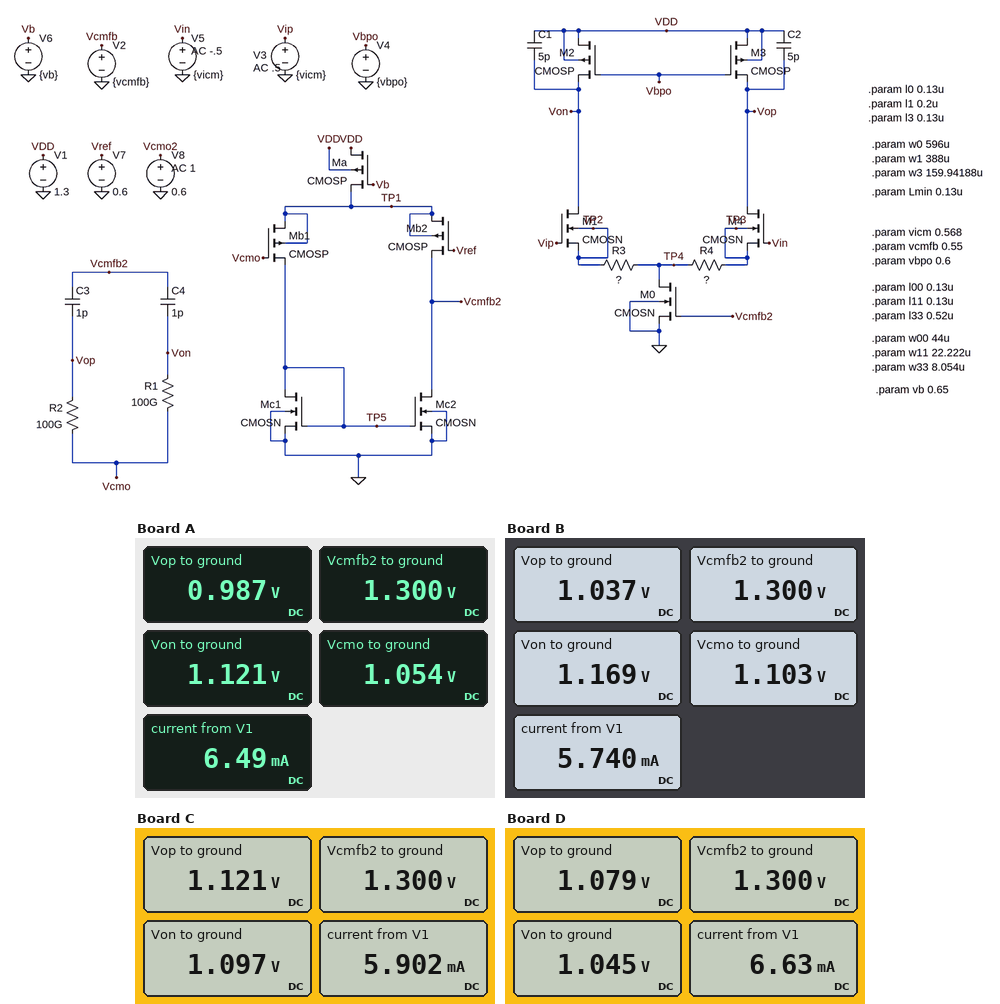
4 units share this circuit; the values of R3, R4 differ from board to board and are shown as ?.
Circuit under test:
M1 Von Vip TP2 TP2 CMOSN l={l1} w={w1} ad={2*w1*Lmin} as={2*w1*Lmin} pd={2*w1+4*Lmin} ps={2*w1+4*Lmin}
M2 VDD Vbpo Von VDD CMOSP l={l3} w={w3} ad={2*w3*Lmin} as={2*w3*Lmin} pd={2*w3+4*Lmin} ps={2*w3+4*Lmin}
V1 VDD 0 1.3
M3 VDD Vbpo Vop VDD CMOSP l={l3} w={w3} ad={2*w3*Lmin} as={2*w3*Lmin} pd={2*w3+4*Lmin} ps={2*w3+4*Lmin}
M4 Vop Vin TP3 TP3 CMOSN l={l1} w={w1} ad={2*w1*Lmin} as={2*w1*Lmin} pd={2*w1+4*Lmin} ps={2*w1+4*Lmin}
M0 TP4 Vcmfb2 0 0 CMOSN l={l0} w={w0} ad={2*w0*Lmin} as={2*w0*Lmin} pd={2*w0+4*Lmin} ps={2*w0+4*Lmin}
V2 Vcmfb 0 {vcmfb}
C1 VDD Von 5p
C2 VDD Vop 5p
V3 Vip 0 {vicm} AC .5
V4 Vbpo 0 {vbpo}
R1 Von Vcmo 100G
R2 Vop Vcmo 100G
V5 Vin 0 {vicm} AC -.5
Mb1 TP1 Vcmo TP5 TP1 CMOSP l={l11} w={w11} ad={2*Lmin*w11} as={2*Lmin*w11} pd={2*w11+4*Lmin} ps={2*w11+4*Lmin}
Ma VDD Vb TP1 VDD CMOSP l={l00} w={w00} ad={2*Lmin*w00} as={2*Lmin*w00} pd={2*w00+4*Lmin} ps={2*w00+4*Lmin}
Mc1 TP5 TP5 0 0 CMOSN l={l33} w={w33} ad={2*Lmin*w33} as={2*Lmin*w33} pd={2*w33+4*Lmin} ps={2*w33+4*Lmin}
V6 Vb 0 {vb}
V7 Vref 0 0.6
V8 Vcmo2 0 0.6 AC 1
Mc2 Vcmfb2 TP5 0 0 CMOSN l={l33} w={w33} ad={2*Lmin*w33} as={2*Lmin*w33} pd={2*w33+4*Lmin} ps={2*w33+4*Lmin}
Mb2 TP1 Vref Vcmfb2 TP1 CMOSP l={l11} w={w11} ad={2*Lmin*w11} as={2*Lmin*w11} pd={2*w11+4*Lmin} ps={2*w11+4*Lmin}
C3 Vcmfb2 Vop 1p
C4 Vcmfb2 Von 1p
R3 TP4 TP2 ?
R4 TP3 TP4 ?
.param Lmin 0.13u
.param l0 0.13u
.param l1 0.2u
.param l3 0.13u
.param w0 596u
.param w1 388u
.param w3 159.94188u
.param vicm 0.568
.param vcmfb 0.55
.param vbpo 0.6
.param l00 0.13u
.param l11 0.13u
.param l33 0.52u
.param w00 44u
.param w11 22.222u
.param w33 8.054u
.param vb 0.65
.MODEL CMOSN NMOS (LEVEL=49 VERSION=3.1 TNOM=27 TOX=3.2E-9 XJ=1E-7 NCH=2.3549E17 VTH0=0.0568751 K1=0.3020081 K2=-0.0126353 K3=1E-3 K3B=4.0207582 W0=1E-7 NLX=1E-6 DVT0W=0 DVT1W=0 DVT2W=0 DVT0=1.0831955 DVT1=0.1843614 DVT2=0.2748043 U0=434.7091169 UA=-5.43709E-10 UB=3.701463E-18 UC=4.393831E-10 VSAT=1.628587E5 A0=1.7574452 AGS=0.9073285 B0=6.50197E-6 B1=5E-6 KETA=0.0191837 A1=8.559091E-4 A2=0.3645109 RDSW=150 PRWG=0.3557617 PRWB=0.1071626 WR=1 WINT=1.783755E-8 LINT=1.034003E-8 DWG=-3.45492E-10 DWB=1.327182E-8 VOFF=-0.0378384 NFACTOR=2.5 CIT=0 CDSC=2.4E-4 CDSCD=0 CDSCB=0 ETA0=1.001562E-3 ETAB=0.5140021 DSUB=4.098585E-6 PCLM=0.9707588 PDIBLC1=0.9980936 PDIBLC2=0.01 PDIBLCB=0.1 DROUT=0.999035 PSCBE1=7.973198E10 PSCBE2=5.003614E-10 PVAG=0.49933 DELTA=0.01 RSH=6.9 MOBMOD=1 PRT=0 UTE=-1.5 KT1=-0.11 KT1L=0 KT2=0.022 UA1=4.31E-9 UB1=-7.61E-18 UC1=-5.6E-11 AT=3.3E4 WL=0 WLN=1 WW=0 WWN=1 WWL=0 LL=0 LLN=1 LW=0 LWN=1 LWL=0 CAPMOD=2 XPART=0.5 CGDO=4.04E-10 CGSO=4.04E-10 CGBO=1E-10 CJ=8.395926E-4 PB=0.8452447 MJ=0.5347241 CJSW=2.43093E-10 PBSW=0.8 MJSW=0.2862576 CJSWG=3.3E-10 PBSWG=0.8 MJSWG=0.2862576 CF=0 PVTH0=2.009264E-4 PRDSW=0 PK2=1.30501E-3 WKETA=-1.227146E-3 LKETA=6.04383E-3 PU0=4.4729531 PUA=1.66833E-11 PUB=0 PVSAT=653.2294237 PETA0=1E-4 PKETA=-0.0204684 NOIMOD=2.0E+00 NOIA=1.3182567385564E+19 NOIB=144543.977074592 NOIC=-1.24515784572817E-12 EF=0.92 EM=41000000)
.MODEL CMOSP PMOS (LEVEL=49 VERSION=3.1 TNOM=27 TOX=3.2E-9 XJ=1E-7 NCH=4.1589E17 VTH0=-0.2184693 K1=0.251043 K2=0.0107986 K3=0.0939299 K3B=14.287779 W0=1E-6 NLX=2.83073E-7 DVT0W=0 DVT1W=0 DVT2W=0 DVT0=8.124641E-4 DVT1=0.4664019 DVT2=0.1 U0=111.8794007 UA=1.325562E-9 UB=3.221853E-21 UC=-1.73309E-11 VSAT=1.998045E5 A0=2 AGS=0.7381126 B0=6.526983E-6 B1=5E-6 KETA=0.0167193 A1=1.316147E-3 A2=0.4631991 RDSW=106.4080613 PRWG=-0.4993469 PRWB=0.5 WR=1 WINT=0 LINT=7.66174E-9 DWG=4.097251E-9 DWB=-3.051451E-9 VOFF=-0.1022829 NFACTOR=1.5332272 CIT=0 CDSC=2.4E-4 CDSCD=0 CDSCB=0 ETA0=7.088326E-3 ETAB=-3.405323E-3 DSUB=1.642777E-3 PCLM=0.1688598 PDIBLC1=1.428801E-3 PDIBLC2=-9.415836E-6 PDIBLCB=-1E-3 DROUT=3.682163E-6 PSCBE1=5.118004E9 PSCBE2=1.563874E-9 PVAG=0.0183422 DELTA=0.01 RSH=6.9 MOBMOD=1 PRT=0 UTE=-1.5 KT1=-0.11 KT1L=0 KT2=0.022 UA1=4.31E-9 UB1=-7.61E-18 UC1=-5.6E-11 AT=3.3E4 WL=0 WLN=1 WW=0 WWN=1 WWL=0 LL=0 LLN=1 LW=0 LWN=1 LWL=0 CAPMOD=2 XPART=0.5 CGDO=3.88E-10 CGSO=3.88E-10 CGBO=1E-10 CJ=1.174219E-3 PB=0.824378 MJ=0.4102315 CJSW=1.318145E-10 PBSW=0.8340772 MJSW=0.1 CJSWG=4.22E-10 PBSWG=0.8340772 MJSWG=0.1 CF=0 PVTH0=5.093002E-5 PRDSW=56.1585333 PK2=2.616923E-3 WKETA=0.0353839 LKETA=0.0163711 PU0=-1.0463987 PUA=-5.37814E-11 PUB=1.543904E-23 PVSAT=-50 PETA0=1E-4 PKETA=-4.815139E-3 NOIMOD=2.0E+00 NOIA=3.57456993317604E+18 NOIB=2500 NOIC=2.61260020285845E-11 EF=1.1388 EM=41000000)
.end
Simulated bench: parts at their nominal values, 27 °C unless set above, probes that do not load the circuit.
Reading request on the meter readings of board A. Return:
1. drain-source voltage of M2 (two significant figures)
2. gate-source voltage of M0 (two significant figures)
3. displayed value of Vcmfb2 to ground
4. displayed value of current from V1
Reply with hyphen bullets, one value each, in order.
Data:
- 180 mV
- 1.3 V
- 1.300 V
- 6.49 mA
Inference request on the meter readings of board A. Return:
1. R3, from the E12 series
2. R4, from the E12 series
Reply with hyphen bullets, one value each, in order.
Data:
- 12 Ω
- 3.3 Ω
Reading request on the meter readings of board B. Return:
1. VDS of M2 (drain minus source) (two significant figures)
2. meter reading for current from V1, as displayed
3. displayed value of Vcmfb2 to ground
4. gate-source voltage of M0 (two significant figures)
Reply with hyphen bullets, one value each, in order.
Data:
- 130 mV
- 5.740 mA
- 1.300 V
- 1.3 V
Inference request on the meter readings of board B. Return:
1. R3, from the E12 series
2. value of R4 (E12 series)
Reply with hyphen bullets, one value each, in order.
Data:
- 27 Ω
- 8.2 Ω
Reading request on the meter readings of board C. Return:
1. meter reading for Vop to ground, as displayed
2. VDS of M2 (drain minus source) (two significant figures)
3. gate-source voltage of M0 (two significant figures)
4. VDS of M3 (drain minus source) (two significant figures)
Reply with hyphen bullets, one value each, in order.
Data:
- 1.121 V
- 200 mV
- 1.3 V
- 180 mV
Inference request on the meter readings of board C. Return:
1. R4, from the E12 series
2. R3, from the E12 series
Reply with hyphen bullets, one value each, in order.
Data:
- 15 Ω
- 12 Ω
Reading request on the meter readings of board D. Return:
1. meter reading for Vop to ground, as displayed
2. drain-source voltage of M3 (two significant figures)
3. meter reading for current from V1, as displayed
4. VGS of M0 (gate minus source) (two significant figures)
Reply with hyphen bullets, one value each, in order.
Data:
- 1.079 V
- 220 mV
- 6.63 mA
- 1.3 V
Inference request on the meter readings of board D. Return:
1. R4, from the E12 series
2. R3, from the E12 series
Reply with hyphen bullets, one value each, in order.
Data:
- 6.8 Ω
- 4.7 Ω
